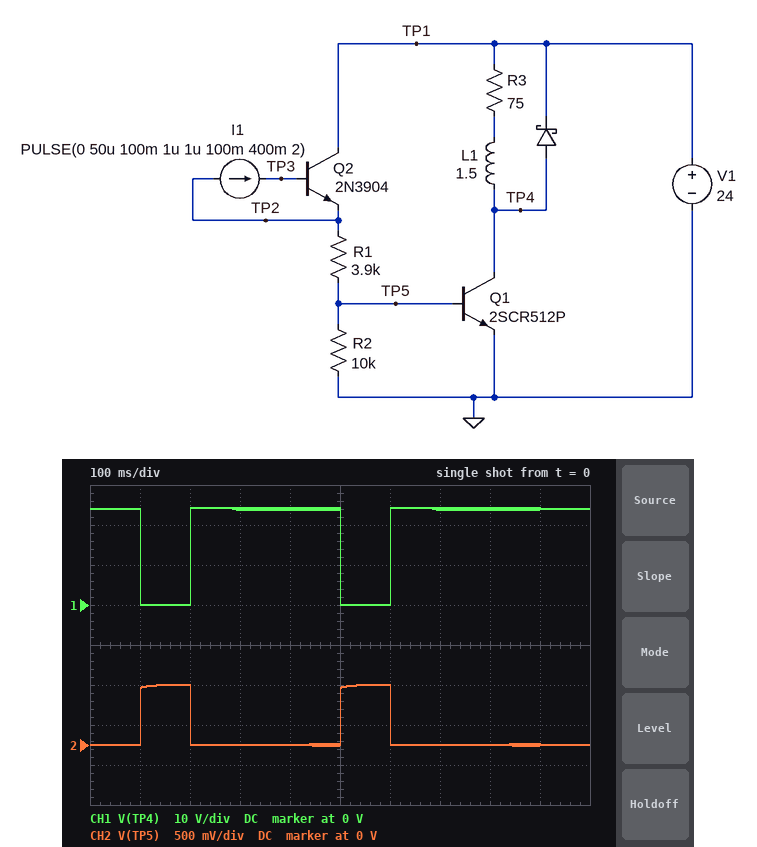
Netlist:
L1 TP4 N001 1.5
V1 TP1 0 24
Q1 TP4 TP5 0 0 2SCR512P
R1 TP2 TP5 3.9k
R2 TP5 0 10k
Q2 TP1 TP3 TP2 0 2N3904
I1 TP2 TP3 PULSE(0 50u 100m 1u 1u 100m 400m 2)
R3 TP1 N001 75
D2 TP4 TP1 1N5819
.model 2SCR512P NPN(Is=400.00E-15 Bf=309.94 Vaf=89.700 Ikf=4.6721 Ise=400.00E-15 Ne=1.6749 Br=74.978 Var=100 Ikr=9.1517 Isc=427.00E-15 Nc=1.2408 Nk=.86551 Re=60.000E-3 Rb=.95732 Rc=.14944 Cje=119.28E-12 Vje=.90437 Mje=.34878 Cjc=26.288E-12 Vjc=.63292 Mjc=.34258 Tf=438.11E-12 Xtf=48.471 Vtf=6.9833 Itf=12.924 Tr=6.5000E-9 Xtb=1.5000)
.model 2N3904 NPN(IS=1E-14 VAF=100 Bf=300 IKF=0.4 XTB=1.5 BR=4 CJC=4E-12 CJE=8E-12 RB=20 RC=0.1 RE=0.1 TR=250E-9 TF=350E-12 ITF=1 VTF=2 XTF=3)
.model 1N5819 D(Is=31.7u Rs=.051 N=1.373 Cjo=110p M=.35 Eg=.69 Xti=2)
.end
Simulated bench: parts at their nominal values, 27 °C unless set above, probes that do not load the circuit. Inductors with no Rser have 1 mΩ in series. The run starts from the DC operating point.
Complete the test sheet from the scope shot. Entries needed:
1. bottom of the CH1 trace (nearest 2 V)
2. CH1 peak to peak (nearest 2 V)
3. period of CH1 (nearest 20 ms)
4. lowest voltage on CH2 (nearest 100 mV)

0 V
24 V
400 ms
0 V
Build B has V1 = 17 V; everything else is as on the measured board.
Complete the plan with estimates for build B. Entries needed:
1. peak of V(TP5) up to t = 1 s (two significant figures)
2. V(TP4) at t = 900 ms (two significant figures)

730 mV
17 V
